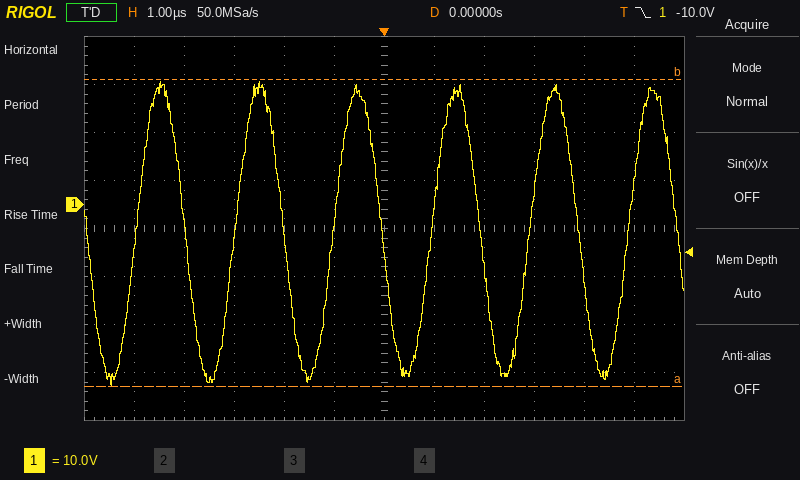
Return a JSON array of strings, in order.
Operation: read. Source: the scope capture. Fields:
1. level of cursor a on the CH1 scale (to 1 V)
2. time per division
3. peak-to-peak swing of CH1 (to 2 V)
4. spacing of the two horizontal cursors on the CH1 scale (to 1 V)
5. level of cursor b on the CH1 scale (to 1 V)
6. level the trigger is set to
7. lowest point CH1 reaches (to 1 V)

["-38 V", "1 µs", "64 V", "64 V", "26 V", "-10.0 V", "-38 V"]
